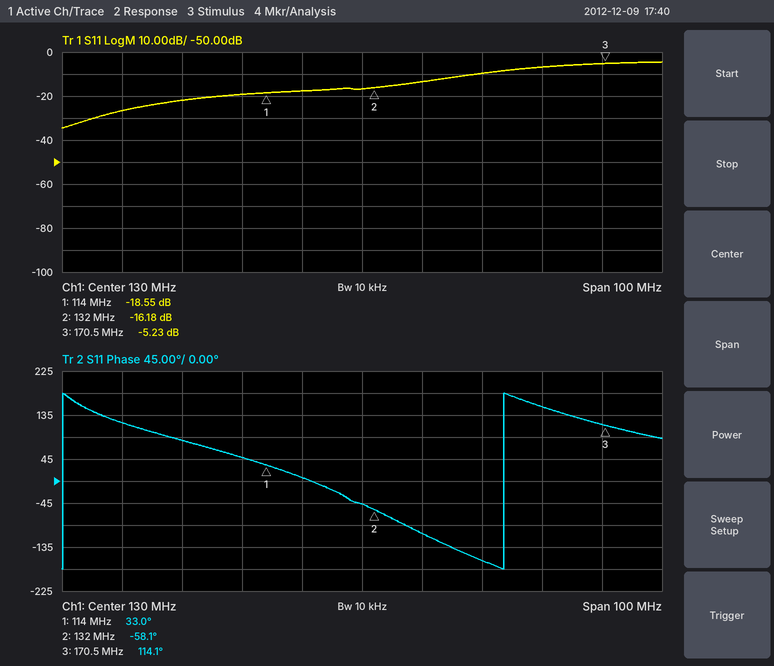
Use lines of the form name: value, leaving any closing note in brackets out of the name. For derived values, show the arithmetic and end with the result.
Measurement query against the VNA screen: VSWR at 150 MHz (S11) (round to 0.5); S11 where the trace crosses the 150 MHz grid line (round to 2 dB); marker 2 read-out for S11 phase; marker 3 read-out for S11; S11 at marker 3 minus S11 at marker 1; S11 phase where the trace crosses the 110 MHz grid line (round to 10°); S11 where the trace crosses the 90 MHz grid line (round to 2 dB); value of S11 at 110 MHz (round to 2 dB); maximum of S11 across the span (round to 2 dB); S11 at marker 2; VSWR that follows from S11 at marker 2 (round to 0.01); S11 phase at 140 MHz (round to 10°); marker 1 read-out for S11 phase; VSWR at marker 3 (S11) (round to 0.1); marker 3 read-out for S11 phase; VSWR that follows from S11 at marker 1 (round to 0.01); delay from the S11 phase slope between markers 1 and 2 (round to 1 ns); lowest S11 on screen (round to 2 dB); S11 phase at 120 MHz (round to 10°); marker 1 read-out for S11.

VSWR at 150 MHz (S11): |Γ| = 10^(-10/20) = 0.3162; VSWR = (1 + 0.3162)/(1 − 0.3162) ≈ 1.92, so 2.0 to the nearest 0.5
S11 where the trace crosses the 150 MHz grid line: -10 dB
marker 2 read-out for S11 phase: -58.1°
marker 3 read-out for S11: -5.23 dB
S11 at marker 3 minus S11 at marker 1: -5.23 − (-18.55) = 13.32 dB
S11 phase where the trace crosses the 110 MHz grid line: 50°
S11 where the trace crosses the 90 MHz grid line: -26 dB
value of S11 at 110 MHz: -20 dB
maximum of S11 across the span: -4 dB
S11 at marker 2: -16.18 dB
VSWR that follows from S11 at marker 2: (1 + 0.1552)/(1 − 0.1552) ≈ 1.37
S11 phase at 140 MHz: -110°
marker 1 read-out for S11 phase: 33.0°
VSWR at marker 3 (S11): (1 + 0.5476)/(1 − 0.5476) ≈ 3.4
marker 3 read-out for S11 phase: 114.1°
VSWR that follows from S11 at marker 1: (1 + 0.1182)/(1 − 0.1182) ≈ 1.27
delay from the S11 phase slope between markers 1 and 2: −(-58.1° − (33°))/(360° × 18 MHz) ≈ 14 ns
lowest S11 on screen: -34 dB
S11 phase at 120 MHz: 10°
marker 1 read-out for S11: -18.55 dB
